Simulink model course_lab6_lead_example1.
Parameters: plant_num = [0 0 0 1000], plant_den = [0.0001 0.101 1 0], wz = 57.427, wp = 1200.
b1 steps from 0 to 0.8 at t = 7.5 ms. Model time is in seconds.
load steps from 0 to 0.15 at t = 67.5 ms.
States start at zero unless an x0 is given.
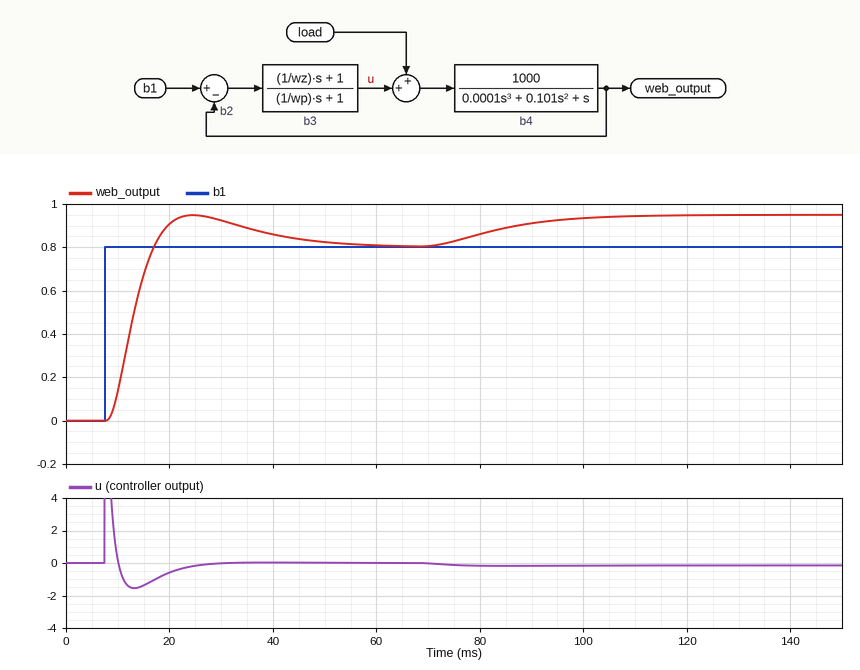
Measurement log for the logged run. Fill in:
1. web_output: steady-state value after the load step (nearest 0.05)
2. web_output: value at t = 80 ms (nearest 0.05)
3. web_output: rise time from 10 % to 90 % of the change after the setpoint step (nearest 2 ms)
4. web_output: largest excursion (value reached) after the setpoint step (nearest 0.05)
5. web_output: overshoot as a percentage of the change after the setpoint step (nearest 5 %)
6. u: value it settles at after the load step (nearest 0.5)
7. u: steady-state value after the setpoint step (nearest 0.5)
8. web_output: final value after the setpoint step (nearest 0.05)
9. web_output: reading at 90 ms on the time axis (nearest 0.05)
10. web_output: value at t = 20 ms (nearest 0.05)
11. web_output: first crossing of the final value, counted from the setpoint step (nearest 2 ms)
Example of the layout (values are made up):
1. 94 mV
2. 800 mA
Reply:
1. 0.95
2. 0.85
3. 6 ms
4. 0.95
5. 20 %
6. 0.0
7. 0.0
8. 0.80
9. 0.90
10. 0.90
11. 10 ms
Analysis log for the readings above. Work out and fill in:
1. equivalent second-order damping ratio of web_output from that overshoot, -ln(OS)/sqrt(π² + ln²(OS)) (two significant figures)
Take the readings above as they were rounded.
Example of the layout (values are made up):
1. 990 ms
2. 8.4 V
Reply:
1. 0.46
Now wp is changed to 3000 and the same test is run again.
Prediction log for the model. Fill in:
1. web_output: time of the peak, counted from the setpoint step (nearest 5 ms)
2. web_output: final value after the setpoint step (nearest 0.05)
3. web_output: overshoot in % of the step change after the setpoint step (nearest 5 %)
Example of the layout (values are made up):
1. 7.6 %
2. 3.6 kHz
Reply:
1. 20 ms
2. 0.80
3. 15 %
